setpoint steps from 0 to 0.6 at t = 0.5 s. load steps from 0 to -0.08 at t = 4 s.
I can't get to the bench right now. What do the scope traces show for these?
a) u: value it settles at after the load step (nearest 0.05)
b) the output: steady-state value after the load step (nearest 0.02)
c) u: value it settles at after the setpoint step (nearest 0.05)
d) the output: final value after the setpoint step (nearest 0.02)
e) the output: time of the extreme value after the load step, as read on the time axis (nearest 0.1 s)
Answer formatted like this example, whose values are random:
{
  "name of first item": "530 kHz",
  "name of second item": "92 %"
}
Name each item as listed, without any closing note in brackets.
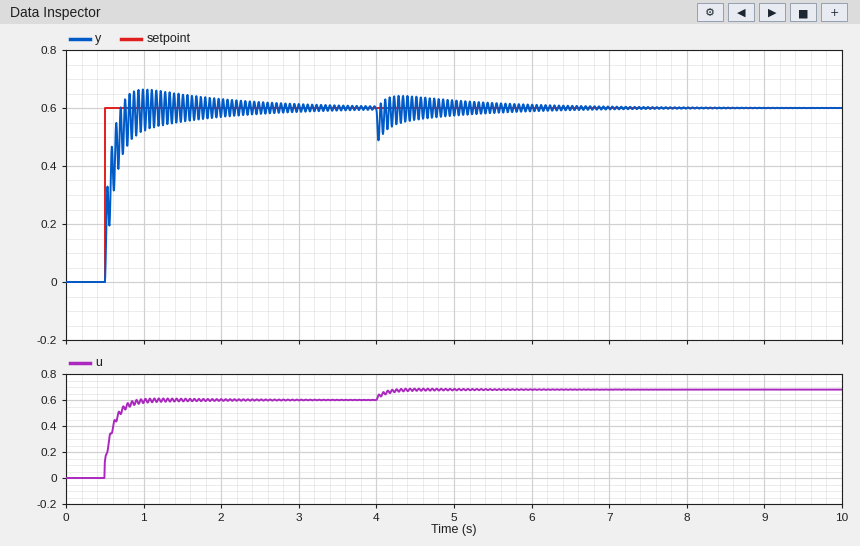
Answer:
{
  "u: value it settles at after the load step": "0.70",
  "the output: steady-state value after the load step": "0.60",
  "u: value it settles at after the setpoint step": "0.60",
  "the output: final value after the setpoint step": "0.60",
  "the output: time of the extreme value after the load step, as read on the time axis": "4.0 s"
}
